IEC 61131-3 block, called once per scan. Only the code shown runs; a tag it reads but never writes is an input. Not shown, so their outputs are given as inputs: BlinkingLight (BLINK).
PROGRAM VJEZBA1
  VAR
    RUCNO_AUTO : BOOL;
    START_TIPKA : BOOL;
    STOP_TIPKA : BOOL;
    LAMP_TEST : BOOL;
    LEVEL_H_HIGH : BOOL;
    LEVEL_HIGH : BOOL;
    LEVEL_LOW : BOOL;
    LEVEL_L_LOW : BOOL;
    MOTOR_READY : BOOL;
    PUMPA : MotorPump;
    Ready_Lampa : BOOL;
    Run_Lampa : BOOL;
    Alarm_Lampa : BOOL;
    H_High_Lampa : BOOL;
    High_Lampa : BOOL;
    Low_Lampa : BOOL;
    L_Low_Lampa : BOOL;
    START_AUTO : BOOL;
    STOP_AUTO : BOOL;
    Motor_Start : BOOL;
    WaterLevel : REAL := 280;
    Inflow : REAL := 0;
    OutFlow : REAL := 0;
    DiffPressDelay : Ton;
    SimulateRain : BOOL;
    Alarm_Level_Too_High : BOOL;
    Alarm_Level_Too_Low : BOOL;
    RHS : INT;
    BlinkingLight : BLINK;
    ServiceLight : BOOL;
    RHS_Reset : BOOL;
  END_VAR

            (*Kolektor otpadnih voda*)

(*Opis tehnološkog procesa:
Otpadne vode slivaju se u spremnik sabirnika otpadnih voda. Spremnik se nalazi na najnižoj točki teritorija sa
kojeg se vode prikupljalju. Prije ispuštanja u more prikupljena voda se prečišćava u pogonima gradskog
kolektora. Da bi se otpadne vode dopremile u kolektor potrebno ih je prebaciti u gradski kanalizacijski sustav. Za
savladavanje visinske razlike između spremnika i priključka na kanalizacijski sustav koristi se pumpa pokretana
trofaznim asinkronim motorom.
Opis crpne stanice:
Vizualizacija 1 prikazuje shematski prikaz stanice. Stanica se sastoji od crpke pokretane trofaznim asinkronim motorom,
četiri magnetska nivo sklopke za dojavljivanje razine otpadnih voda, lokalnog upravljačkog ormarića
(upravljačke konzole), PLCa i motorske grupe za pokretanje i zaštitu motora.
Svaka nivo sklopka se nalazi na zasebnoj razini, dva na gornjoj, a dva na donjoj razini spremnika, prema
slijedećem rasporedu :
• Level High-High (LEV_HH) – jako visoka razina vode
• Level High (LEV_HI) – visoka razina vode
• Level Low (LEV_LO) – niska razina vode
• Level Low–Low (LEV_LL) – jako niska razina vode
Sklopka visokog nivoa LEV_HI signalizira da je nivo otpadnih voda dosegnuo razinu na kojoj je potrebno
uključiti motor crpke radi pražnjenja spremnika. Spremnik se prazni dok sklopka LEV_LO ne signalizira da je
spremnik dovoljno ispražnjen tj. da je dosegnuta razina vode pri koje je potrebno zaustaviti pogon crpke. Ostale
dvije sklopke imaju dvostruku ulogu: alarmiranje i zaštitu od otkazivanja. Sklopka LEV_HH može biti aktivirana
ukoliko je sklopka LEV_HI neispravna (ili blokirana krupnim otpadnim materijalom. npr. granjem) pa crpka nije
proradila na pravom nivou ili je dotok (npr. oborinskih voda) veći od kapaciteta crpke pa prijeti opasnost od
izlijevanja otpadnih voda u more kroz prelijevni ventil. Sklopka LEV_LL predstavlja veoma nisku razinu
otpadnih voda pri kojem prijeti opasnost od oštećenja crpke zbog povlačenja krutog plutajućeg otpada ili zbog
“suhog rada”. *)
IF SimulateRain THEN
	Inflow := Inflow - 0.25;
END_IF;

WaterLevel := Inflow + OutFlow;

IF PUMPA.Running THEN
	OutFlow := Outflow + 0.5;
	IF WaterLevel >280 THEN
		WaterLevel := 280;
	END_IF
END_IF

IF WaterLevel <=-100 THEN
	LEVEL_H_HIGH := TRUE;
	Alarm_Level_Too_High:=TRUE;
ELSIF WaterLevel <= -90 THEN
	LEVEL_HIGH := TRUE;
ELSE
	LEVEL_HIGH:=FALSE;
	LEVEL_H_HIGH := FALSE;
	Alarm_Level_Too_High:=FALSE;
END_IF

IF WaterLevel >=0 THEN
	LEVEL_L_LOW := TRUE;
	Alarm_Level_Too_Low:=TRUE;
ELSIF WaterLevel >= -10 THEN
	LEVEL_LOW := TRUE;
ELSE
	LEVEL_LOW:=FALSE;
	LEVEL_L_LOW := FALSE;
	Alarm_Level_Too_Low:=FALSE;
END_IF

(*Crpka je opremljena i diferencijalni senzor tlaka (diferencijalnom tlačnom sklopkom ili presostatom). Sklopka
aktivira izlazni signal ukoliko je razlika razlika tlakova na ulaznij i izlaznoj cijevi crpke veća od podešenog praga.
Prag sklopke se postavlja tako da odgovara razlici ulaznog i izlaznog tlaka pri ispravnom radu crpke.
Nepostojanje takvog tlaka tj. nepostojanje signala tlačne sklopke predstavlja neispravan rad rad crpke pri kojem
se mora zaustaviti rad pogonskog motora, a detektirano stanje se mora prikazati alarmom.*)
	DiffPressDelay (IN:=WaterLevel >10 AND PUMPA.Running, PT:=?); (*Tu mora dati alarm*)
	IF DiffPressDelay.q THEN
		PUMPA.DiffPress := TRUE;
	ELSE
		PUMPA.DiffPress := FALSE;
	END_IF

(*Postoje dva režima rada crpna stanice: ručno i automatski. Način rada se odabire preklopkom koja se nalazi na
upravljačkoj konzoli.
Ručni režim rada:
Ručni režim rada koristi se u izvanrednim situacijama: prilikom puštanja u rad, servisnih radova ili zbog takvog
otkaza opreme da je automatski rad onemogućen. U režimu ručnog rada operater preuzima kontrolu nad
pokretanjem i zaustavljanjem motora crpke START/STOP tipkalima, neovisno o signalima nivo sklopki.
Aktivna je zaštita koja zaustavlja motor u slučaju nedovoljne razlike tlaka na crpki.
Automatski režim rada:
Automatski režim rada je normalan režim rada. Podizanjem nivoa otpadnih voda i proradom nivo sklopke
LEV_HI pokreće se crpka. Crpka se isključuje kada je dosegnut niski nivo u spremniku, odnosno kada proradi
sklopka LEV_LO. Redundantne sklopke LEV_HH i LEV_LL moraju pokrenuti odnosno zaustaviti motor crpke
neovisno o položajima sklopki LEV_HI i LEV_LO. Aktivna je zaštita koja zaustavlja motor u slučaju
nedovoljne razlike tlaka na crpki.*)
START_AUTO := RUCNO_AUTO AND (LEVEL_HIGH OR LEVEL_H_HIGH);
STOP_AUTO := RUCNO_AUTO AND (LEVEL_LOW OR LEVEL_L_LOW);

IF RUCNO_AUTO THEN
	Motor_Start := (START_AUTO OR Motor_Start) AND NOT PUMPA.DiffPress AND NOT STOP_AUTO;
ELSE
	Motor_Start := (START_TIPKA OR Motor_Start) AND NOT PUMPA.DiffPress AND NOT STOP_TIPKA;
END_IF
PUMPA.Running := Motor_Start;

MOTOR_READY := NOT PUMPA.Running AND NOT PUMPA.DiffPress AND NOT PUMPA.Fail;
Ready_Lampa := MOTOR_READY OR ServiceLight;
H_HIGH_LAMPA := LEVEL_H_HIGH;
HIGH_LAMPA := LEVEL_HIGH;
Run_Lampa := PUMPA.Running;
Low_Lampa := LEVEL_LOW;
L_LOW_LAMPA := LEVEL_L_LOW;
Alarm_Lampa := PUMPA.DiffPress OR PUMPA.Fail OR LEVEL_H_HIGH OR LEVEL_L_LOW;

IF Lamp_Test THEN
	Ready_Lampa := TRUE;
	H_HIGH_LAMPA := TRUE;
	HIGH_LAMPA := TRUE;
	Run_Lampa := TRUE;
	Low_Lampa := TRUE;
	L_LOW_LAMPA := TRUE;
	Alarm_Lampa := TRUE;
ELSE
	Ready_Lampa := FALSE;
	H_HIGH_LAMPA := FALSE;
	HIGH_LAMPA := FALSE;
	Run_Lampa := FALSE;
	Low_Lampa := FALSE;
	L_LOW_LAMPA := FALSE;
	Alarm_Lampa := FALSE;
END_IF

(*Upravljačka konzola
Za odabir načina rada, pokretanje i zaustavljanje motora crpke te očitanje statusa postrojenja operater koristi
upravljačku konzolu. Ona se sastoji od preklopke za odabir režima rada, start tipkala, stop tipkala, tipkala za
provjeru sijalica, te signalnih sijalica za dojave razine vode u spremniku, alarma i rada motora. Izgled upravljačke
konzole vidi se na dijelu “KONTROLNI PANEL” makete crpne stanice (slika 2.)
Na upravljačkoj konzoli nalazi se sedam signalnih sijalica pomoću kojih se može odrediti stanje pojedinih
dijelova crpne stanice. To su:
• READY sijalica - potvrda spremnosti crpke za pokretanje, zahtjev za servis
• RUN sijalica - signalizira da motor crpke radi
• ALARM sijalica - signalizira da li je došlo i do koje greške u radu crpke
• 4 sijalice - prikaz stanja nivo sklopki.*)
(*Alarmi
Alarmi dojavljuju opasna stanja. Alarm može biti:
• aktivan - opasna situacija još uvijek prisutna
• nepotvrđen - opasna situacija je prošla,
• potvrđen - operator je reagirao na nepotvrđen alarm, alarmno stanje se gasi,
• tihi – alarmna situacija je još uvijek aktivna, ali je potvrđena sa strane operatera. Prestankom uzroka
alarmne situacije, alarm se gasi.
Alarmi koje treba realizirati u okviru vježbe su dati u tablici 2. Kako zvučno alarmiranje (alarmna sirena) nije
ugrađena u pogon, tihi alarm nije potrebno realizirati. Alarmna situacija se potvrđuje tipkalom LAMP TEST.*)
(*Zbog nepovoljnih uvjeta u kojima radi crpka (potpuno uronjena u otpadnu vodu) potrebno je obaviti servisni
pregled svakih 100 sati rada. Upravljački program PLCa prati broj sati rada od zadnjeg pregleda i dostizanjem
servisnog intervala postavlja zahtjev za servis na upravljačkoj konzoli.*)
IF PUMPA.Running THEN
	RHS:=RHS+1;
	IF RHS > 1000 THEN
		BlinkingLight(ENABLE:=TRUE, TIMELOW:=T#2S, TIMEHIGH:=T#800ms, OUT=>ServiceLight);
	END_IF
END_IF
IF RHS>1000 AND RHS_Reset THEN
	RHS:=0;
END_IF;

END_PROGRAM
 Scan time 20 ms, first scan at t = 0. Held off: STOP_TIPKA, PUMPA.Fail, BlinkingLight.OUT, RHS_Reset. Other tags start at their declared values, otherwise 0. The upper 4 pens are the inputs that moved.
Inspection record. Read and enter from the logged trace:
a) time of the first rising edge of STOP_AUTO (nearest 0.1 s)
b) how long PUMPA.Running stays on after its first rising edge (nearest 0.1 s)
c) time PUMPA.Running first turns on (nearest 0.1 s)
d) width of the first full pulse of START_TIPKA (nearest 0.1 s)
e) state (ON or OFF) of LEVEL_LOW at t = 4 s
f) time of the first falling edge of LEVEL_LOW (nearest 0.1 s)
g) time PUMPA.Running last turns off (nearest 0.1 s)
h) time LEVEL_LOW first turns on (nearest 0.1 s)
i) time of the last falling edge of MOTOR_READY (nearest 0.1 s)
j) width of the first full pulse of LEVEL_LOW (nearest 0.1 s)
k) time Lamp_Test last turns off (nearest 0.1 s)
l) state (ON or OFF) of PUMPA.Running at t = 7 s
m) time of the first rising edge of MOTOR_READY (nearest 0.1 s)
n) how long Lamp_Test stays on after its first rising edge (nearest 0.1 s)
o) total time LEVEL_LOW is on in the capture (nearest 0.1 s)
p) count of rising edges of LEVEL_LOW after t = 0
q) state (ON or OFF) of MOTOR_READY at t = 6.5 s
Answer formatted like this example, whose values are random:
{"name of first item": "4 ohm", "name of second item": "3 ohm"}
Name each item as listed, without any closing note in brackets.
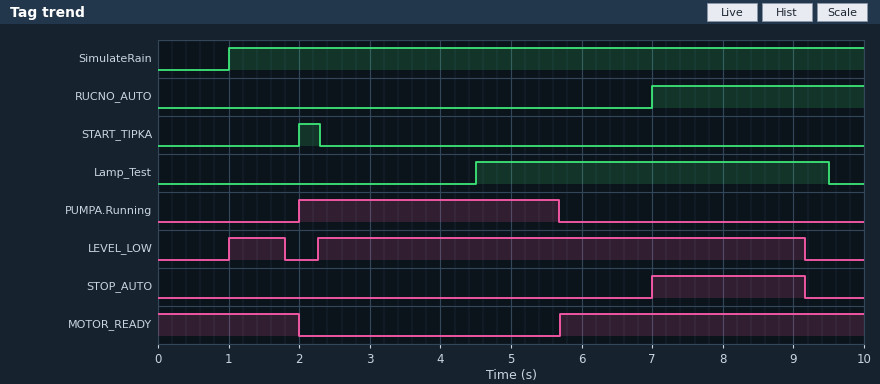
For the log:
{"time of the first rising edge of STOP_AUTO": "7.0 s", "how long PUMPA.Running stays on after its first rising edge": "3.7 s", "time PUMPA.Running first turns on": "2.0 s", "width of the first full pulse of START_TIPKA": "0.3 s", "state (ON or OFF) of LEVEL_LOW at t = 4 s": "ON", "time of the first falling edge of LEVEL_LOW": "1.8 s", "time PUMPA.Running last turns off": "5.7 s", "time LEVEL_LOW first turns on": "1.0 s", "time of the last falling edge of MOTOR_READY": "2.0 s", "width of the first full pulse of LEVEL_LOW": "0.8 s", "time Lamp_Test last turns off": "9.5 s", "state (ON or OFF) of PUMPA.Running at t = 7 s": "OFF", "time of the first rising edge of MOTOR_READY": "5.7 s", "how long Lamp_Test stays on after its first rising edge": "5.0 s", "total time LEVEL_LOW is on in the capture": "7.7 s", "count of rising edges of LEVEL_LOW after t = 0": "2", "state (ON or OFF) of MOTOR_READY at t = 6.5 s": "ON"}
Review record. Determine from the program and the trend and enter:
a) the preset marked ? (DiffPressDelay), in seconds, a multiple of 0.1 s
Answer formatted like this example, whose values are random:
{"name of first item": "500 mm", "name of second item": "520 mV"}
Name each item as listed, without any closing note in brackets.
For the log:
{"the preset marked ? (DiffPressDelay), in seconds, a multiple of 0.1 s": "1.8 s"}
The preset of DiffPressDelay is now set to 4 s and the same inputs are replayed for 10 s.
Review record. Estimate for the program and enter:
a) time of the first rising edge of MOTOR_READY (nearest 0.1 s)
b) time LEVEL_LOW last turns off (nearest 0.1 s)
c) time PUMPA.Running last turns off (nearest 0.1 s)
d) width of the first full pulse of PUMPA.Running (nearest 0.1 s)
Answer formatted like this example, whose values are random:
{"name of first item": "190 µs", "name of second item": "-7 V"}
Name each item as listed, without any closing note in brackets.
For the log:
{"time of the first rising edge of MOTOR_READY": "7.0 s", "time LEVEL_LOW last turns off": "1.8 s", "time PUMPA.Running last turns off": "7.0 s", "width of the first full pulse of PUMPA.Running": "5.0 s"}
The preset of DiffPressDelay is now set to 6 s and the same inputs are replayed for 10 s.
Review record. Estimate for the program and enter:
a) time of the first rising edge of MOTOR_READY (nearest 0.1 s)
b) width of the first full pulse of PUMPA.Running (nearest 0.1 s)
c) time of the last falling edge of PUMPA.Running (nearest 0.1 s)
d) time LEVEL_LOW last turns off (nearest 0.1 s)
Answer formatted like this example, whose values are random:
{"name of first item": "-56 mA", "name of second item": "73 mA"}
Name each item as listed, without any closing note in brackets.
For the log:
{"time of the first rising edge of MOTOR_READY": "7.0 s", "width of the first full pulse of PUMPA.Running": "5.0 s", "time of the last falling edge of PUMPA.Running": "7.0 s", "time LEVEL_LOW last turns off": "1.8 s"}
